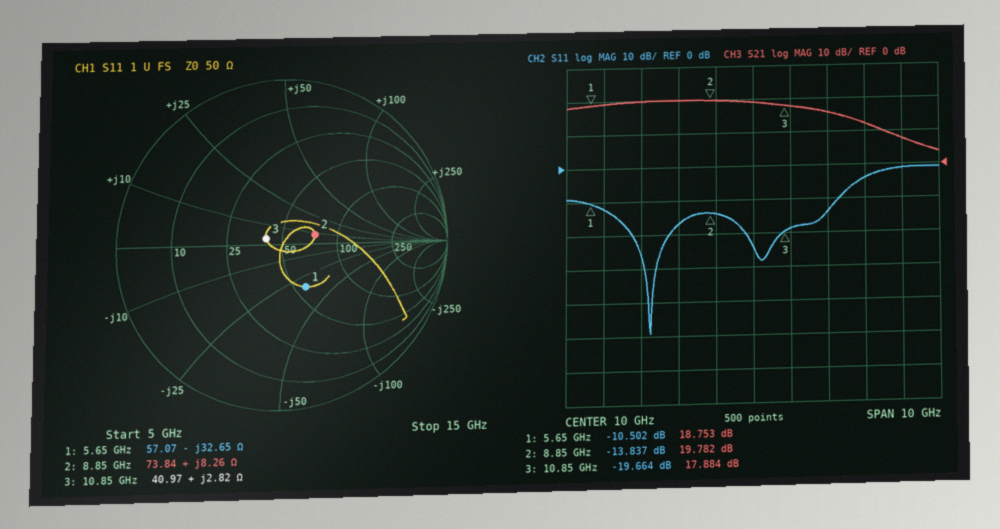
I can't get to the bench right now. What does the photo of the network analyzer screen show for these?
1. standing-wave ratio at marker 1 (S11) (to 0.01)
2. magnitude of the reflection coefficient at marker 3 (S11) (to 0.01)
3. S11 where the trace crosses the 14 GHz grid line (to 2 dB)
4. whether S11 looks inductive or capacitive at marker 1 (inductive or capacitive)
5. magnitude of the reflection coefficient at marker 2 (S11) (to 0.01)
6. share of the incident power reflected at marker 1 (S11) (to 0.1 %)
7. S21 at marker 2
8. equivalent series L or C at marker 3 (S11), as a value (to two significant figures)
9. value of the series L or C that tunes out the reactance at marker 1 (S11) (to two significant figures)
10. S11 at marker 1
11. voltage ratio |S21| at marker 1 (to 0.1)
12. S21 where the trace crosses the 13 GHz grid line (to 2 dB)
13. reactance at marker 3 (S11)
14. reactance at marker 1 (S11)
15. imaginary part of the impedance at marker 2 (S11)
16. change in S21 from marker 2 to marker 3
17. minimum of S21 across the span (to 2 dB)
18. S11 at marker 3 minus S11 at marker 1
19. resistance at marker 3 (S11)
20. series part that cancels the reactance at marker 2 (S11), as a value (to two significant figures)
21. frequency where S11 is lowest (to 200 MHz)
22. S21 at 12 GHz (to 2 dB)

1.85
0.10
-2 dB
capacitive
0.20
8.9 %
19.782 dB
41 pH
920 pH
-10.502 dB
8.7
12 dB
+2.82 Ω
-32.65 Ω
+8.26 Ω
-1.898 dB
4 dB
-9.162 dB
40.97 Ω
2.2 pF
7.2 GHz
16 dB
